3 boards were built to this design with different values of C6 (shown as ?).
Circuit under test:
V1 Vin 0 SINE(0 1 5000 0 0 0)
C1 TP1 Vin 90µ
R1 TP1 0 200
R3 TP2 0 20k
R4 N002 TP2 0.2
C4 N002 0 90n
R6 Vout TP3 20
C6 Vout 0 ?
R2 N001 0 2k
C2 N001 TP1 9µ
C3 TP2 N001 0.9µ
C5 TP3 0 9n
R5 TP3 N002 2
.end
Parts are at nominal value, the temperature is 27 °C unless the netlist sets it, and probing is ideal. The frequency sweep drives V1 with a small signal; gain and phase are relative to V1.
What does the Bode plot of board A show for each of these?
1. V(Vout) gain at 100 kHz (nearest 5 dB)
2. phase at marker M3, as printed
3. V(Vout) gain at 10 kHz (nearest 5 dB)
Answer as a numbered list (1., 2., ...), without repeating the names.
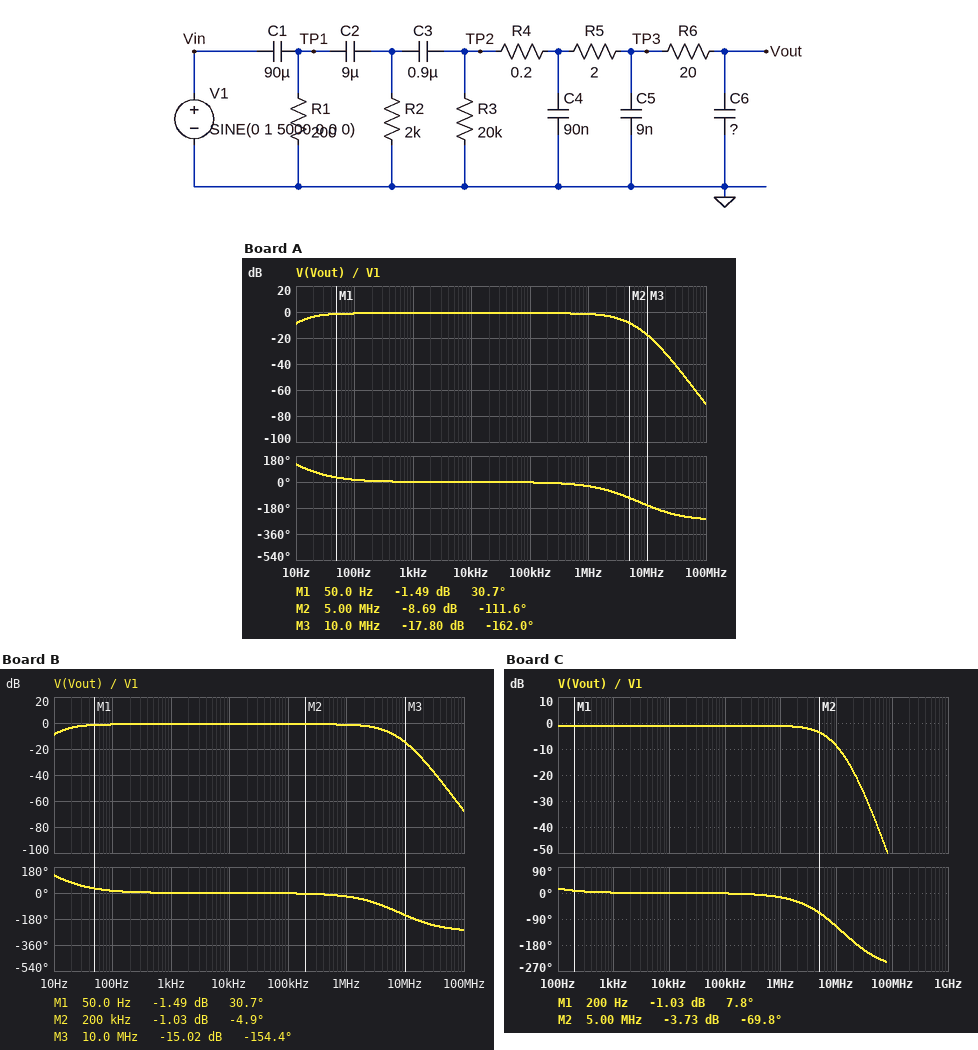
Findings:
1. 0 dB
2. -162.0 deg
3. 0 dB
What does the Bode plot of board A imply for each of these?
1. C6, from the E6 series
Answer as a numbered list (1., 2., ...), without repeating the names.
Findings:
1. 2.2 nF
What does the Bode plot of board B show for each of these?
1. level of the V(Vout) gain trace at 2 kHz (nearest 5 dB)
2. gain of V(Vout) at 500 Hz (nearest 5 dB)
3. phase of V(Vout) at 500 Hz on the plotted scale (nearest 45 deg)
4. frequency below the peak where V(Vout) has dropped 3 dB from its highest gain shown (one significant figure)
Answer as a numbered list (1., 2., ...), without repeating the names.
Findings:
1. 0 dB
2. 0 dB
3. 0 deg
4. 20 Hz
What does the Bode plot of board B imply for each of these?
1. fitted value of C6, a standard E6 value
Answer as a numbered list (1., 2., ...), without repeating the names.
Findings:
1. 1.5 nF
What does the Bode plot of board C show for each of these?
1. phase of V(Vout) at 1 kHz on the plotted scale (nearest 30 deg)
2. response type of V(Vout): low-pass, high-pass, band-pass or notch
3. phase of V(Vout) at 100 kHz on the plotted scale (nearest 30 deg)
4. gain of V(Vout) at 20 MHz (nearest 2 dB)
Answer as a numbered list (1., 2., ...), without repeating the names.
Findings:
1. 0 deg
2. low-pass
3. 0 deg
4. -18 dB
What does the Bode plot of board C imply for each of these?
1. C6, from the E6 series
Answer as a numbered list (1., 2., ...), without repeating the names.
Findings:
1. 330 pF
